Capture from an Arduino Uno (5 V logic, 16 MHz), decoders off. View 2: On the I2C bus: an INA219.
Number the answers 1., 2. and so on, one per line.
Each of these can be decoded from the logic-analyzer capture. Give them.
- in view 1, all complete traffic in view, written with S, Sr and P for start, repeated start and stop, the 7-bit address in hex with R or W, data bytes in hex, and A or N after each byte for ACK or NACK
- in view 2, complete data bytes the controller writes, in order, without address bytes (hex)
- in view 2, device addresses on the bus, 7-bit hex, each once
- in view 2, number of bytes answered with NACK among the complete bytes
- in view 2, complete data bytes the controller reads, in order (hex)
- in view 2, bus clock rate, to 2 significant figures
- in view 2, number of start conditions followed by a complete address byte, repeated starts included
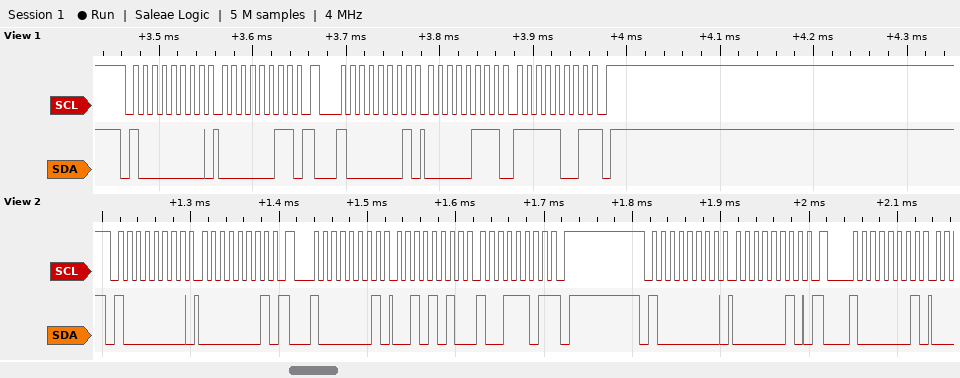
1. S 40W A 03 A Sr 40R A 07 A F9 N P
2. 01 02
3. 0x40
4. 1
5. 2A 9D
6. 100 kHz
7. 4
